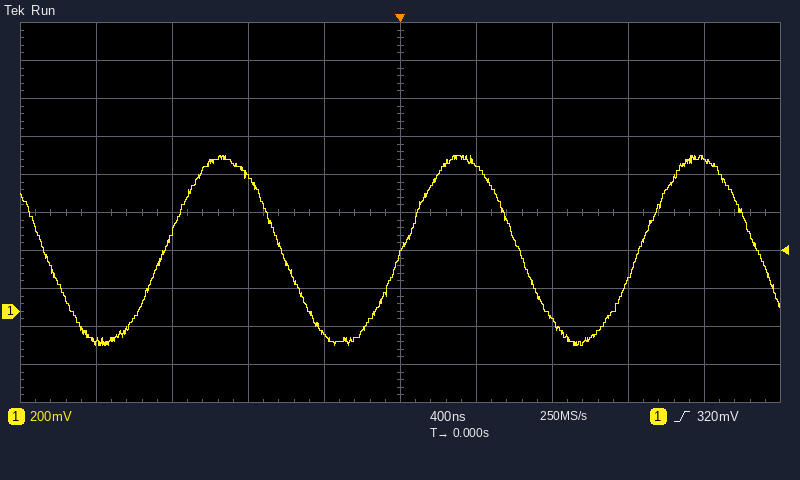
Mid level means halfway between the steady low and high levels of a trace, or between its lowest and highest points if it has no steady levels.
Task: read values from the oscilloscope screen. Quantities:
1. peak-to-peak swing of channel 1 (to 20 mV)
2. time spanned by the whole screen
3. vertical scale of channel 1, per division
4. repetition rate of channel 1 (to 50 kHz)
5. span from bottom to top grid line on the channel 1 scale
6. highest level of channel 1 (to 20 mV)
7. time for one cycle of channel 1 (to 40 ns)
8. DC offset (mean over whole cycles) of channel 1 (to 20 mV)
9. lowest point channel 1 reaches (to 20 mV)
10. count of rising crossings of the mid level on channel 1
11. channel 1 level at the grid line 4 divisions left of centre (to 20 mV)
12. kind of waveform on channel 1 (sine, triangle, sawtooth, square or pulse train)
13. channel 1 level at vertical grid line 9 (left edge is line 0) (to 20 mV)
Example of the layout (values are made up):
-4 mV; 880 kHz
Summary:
1.00 V; 4 µs; 200 mV; 800 kHz; 2 V; 820 mV; 1.24 µs; 320 mV; -180 mV; 3; -160 mV; sine; 800 mV
